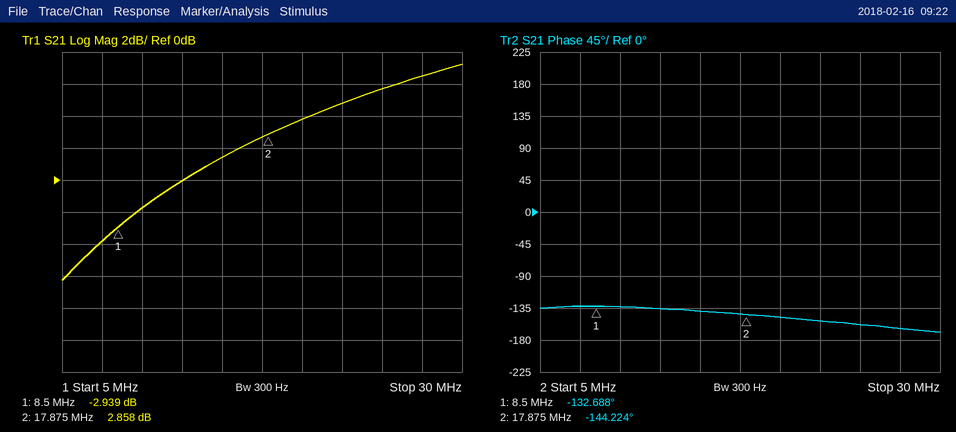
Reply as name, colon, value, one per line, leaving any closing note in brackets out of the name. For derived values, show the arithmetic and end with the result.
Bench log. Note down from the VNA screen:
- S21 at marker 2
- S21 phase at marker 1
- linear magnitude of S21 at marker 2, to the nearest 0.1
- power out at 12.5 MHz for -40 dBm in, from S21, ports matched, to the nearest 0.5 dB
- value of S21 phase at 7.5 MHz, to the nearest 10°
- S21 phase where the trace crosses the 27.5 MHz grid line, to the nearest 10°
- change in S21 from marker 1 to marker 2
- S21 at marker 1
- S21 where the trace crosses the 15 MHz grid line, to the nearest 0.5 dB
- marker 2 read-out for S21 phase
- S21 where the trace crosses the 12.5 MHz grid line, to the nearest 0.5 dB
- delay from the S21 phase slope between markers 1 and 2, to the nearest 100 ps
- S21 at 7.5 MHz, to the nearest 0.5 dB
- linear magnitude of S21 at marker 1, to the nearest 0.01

S21 at marker 2: 2.858 dB
S21 phase at marker 1: -132.688°
linear magnitude of S21 at marker 2, to the nearest 0.1: 10^(2.858/20) ≈ 1.4
power out at 12.5 MHz for -40 dBm in, from S21, ports matched, to the nearest 0.5 dB: -40 dBm + (0.0 dB) = -40.0 dBm
value of S21 phase at 7.5 MHz, to the nearest 10°: -130°
S21 phase where the trace crosses the 27.5 MHz grid line, to the nearest 10°: -160°
change in S21 from marker 1 to marker 2: 2.858 − (-2.939) = 5.797 dB
S21 at marker 1: -2.939 dB
S21 where the trace crosses the 15 MHz grid line, to the nearest 0.5 dB: 1.5 dB
marker 2 read-out for S21 phase: -144.224°
S21 where the trace crosses the 12.5 MHz grid line, to the nearest 0.5 dB: 0.0 dB
delay from the S21 phase slope between markers 1 and 2, to the nearest 100 ps: −(-144.224° − (-132.688°))/(360° × 9.375 MHz) ≈ 3.4 ns
S21 at 7.5 MHz, to the nearest 0.5 dB: -4.0 dB
linear magnitude of S21 at marker 1, to the nearest 0.01: 10^(-2.939/20) ≈ 0.71
